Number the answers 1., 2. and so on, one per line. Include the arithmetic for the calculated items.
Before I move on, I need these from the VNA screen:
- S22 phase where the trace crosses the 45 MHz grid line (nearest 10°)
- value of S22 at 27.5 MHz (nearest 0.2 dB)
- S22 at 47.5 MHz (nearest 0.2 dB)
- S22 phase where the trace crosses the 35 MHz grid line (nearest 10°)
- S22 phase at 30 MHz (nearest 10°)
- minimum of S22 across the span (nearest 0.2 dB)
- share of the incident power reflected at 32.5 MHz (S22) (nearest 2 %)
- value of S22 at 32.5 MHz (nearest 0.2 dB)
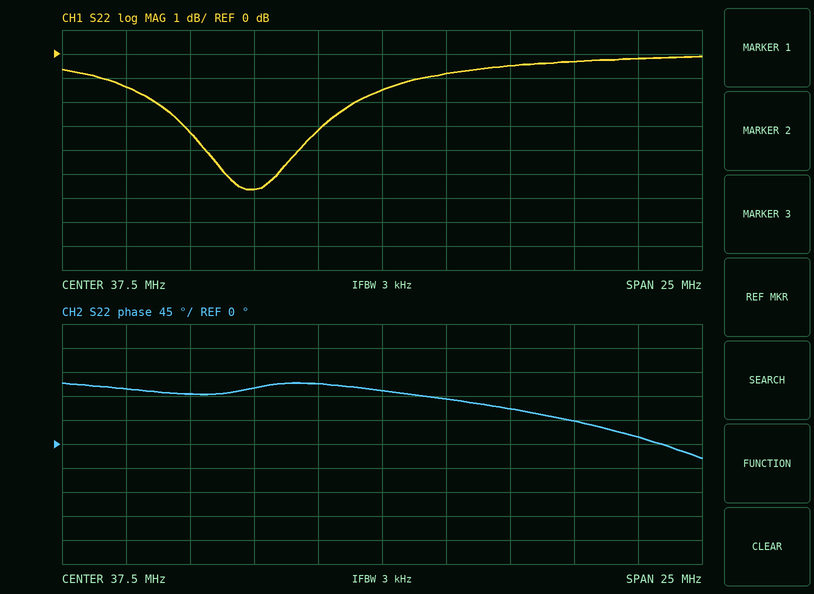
1. 40°
2. -1.4 dB
3. -0.2 dB
4. 110°
5. 90°
6. -5.6 dB
7. 10^(-5.6/10) ≈ 28 %
8. -5.6 dB
